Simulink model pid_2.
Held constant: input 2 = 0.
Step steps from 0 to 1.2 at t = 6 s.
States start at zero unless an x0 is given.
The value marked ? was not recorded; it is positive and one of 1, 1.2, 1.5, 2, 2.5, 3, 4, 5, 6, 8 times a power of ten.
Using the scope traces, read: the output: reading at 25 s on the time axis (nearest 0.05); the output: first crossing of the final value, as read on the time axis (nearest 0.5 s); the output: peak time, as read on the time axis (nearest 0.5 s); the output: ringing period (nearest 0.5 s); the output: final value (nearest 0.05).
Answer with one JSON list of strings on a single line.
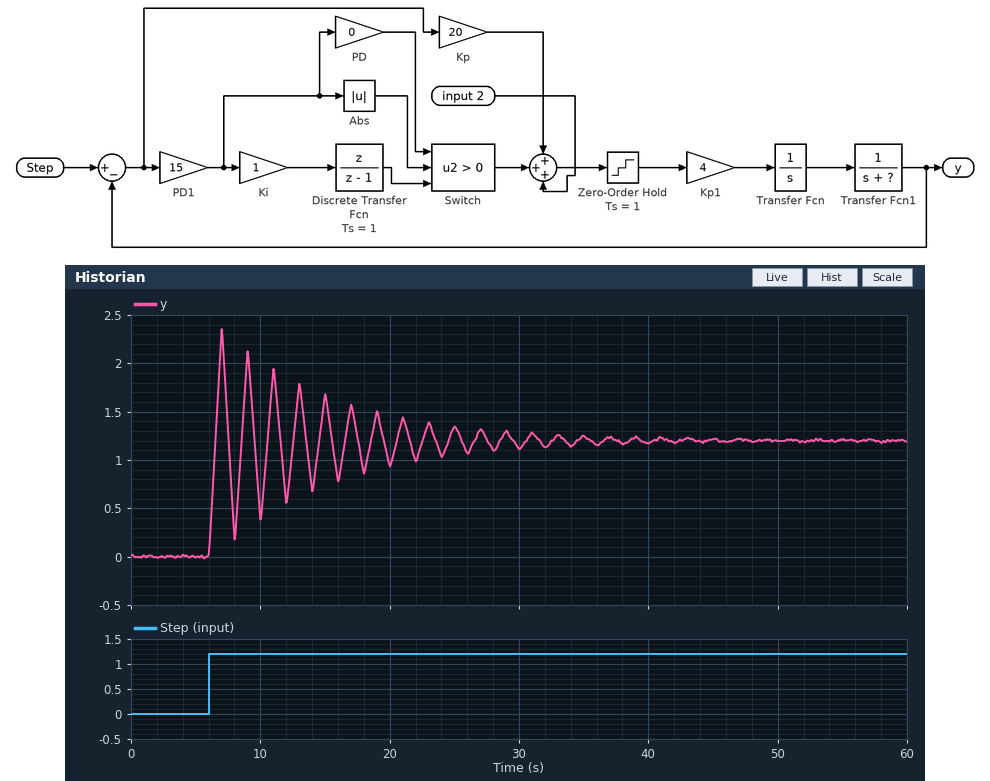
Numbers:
["1.35", "6.5 s", "7.0 s", "2.0 s", "1.20"]
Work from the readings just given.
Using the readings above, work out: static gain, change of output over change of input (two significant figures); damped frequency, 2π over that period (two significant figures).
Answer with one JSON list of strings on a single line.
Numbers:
["1.0", "3.1 rad/s"]
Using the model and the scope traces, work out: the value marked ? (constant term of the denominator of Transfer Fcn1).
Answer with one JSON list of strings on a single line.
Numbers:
["40"]
